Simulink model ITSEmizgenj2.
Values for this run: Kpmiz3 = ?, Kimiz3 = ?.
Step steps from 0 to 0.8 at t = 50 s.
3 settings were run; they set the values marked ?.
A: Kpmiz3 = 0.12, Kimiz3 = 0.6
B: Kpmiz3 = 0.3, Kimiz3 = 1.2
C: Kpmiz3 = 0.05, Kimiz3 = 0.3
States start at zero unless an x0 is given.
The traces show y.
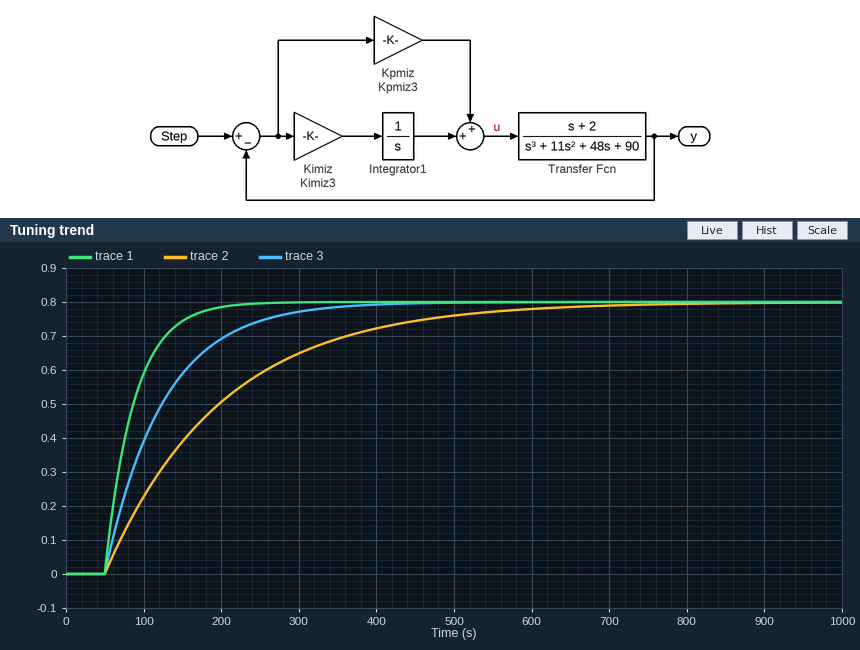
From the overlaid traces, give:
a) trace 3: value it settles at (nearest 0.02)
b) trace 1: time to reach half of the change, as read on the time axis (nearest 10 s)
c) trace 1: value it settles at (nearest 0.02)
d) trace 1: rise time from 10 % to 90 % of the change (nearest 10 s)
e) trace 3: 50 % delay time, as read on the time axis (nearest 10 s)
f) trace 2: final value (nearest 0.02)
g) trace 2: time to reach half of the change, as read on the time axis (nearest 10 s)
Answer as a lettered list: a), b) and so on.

a) 0.80
b) 80 s
c) 0.80
d) 80 s
e) 100 s
f) 0.80
g) 150 s
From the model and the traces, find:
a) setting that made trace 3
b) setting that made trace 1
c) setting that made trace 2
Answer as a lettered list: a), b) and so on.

a) A
b) B
c) C
